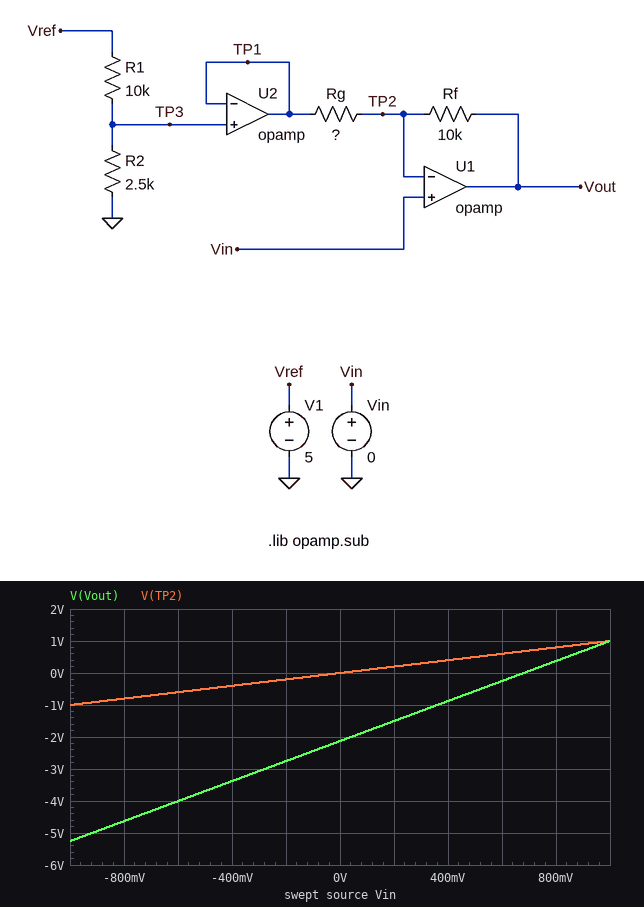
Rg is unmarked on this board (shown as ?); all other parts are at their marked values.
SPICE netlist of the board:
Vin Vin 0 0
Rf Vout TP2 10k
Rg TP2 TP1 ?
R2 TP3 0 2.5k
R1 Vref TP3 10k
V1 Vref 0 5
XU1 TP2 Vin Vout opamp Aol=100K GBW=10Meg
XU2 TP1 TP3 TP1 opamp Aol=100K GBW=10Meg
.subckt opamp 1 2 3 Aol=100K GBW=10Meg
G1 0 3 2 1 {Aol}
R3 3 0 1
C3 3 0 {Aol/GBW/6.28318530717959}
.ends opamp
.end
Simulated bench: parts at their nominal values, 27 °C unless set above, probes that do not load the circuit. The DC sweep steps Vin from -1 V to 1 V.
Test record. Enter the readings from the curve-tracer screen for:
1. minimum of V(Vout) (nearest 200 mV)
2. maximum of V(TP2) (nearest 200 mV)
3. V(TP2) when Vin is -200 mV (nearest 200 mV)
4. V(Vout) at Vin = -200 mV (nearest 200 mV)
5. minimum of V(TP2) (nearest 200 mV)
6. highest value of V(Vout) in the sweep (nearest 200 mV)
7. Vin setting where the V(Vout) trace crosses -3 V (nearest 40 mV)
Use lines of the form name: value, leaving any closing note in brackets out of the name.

minimum of V(Vout): -5.2 V
maximum of V(TP2): 1.0 V
V(TP2) when Vin is -200 mV: -200 mV
V(Vout) at Vin = -200 mV: -2.8 V
minimum of V(TP2): -1.0 V
highest value of V(Vout) in the sweep: 1.0 V
Vin setting where the V(Vout) trace crosses -3 V: -280 mV
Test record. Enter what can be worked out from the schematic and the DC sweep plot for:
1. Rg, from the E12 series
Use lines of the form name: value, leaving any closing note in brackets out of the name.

Rg, from the E12 series: 4.7 kΩ
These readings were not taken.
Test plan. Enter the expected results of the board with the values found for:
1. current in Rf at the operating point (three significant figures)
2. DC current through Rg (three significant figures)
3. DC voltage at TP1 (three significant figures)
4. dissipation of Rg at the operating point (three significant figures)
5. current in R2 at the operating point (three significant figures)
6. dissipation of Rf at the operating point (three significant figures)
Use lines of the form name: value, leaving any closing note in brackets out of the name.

current in Rf at the operating point: 213 µA
DC current through Rg: 213 µA
DC voltage at TP1: 1.00 V
dissipation of Rg at the operating point: 213 µW
current in R2 at the operating point: 400 µA
dissipation of Rf at the operating point: 453 µW
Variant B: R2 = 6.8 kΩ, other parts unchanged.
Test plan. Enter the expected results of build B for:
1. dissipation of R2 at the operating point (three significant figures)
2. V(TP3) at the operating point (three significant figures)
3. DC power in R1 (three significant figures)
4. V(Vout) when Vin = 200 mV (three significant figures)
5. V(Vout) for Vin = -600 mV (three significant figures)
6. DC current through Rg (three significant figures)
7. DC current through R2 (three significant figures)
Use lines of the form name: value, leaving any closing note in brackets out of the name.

dissipation of R2 at the operating point: 602 µW
V(TP3) at the operating point: 2.02 V
DC power in R1: 886 µW
V(Vout) when Vin = 200 mV: -3.68 V
V(Vout) for Vin = -600 mV: -6.18 V
DC current through Rg: 431 µA
DC current through R2: 298 µA
